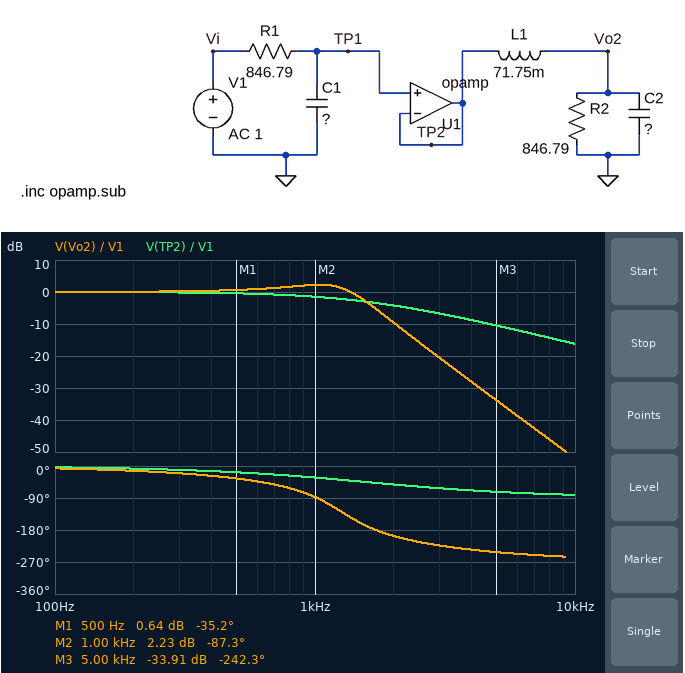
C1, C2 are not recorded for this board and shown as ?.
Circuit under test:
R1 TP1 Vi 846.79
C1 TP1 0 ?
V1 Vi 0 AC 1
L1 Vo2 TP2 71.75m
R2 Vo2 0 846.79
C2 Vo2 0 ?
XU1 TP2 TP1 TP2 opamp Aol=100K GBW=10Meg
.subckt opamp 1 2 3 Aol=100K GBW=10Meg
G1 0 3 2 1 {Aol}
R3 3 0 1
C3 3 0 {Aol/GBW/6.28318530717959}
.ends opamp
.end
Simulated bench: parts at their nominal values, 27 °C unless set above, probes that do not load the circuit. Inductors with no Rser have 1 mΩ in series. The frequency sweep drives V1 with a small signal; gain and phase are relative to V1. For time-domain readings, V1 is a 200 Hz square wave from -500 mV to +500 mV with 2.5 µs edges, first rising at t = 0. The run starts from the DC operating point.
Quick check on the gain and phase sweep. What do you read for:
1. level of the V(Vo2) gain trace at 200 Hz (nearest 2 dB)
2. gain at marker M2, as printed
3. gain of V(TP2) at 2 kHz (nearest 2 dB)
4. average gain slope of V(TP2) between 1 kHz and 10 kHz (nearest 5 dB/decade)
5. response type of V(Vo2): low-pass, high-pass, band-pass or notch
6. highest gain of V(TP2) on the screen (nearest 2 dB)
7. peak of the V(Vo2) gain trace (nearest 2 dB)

0 dB
2.23 dB
-4 dB
-15 dB/decade
low-pass
0 dB
2 dB
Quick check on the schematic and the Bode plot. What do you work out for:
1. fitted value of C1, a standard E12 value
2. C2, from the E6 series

120 nF
220 nF
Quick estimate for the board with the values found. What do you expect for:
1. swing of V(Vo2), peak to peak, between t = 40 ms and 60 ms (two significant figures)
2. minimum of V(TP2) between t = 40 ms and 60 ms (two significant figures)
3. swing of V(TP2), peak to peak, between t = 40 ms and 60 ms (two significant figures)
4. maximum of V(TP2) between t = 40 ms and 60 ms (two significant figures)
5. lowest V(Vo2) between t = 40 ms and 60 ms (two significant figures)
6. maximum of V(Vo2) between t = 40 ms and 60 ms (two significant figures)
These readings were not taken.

1.5 V
-500 mV
1.0 V
500 mV
-730 mV
730 mV
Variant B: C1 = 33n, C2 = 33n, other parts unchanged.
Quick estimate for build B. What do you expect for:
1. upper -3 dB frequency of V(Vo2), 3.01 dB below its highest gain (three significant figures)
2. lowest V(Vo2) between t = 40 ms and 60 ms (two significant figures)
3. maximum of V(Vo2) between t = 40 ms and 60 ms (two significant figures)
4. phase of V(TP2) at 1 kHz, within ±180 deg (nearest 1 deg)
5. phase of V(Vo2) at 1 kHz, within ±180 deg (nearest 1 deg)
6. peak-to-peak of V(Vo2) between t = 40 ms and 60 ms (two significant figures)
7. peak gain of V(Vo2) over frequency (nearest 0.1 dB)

2.27 kHz
-500 mV
500 mV
-10 deg
-40 deg
1.0 V
0 dB
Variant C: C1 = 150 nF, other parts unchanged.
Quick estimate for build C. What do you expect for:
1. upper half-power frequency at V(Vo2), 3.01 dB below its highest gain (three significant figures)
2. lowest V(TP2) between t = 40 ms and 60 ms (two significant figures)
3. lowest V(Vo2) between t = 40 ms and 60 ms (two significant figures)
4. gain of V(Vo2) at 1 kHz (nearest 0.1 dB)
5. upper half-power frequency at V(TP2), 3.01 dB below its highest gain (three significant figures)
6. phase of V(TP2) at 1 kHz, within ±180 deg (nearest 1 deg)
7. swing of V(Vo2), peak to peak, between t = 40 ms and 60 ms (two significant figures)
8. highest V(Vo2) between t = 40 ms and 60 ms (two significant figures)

1.41 kHz
-500 mV
-690 mV
1.6 dB
1.25 kHz
-39 deg
1.4 V
690 mV
